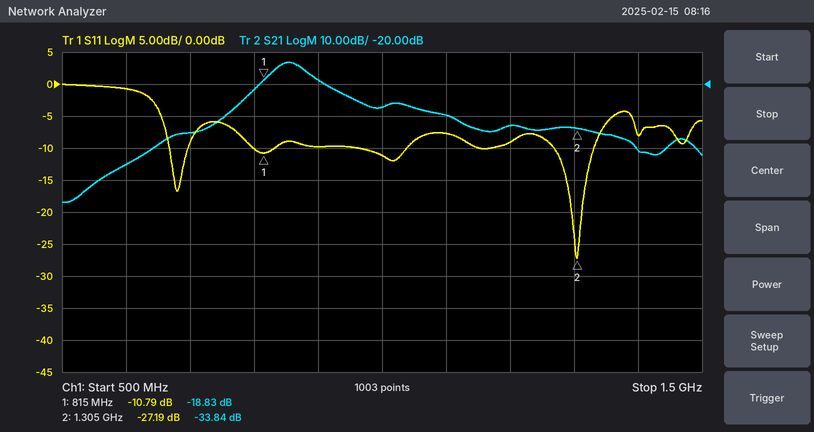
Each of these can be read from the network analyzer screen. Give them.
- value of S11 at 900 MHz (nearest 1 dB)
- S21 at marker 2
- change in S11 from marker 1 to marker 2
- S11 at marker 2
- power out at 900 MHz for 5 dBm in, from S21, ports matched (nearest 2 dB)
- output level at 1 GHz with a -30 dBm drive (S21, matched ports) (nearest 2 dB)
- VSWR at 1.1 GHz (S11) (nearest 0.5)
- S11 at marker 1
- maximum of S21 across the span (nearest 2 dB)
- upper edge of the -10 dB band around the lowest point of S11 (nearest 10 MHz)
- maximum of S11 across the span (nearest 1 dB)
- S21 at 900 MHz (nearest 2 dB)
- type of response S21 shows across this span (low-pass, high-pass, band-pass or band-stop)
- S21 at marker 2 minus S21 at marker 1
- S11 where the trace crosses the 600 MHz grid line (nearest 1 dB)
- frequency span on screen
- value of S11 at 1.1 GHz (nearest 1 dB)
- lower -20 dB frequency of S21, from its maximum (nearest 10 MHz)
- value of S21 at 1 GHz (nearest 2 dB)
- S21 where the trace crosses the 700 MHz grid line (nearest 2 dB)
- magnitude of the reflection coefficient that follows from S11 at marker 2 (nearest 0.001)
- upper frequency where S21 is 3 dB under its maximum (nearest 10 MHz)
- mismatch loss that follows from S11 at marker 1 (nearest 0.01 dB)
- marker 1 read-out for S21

-10 dB
-33.84 dB
-16.40 dB
-27.19 dB
-14 dBm
-58 dBm
2.5
-10.79 dB
-14 dB
1.33 GHz
0 dB
-18 dB
band-pass
-15.01 dB
-1 dB
1 GHz
-8 dB
730 MHz
-28 dB
-36 dB
0.044
880 MHz
0.38 dB
-18.83 dB
